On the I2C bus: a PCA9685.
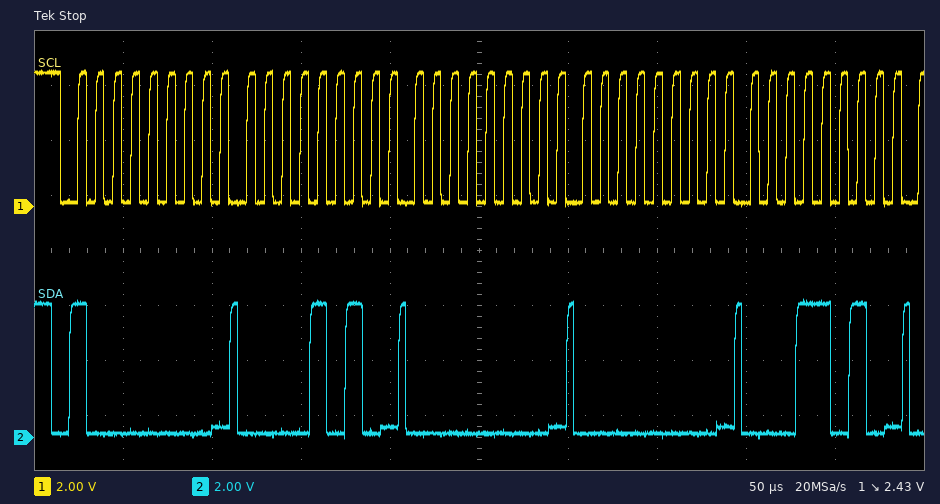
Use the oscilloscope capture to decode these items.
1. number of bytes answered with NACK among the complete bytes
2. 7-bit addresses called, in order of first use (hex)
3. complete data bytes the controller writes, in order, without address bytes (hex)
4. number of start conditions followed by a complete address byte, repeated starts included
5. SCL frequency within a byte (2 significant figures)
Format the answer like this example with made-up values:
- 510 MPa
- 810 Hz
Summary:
- 0
- 0x40
- 0A 00 00 1A
- 1
- 100 kHz
